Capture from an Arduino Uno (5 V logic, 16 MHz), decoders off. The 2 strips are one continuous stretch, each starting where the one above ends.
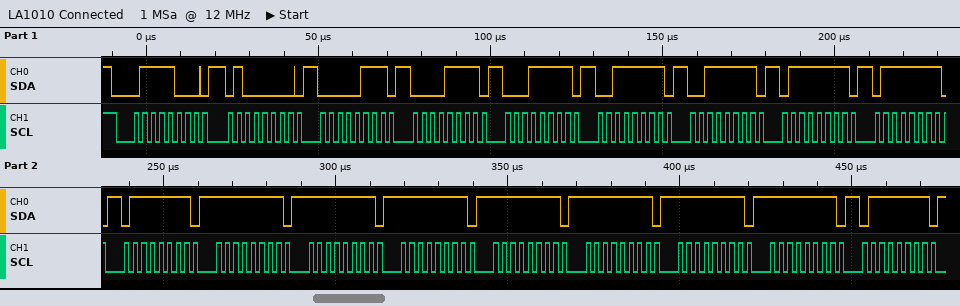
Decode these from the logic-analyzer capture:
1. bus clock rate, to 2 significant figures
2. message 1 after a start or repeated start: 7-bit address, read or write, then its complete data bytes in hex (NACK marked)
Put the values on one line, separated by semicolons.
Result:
400 kHz; 0x3C write: 40 07 0F 1F 3F 3F 7F 7F 7F FF FF FF FF FF FF FF 7F
